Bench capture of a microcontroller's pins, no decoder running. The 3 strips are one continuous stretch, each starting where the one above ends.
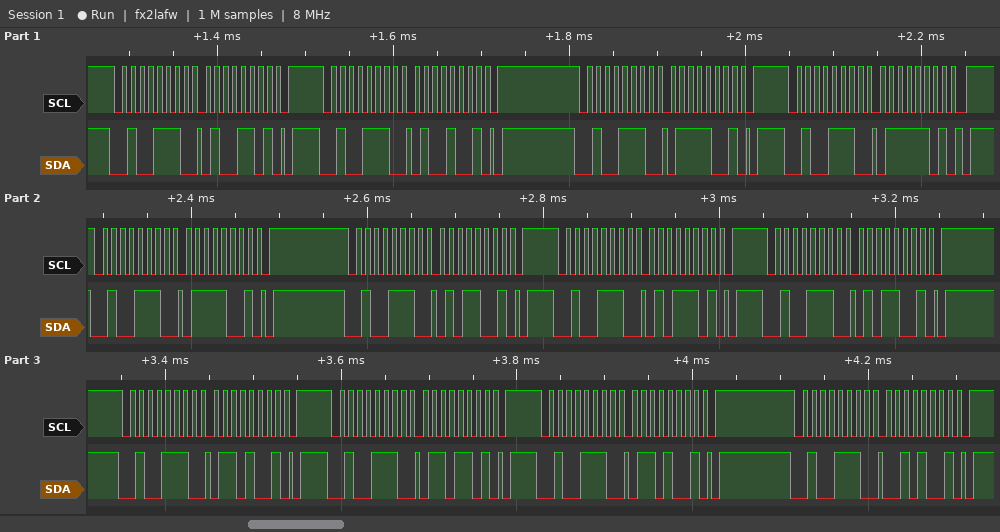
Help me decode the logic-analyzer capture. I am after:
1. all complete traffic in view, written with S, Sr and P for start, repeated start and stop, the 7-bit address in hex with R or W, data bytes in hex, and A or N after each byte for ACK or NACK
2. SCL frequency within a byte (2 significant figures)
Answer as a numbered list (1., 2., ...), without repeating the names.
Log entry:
1. S 27W A 4D A P S 27W A 49 A P S 27W A 79 A P S 27W A 7D A P S 27W A 79 A P S 27W A 59 A P S 27W A 5D A P S 27W A 59 A P S 27W A 69 A P S 27W A 6D A P S 27W A 69 A P S 27W A 29 A P
2. 100 kHz
